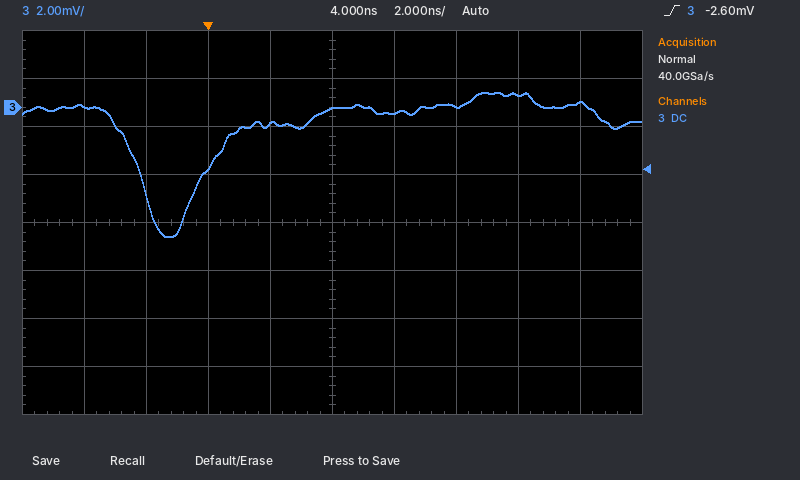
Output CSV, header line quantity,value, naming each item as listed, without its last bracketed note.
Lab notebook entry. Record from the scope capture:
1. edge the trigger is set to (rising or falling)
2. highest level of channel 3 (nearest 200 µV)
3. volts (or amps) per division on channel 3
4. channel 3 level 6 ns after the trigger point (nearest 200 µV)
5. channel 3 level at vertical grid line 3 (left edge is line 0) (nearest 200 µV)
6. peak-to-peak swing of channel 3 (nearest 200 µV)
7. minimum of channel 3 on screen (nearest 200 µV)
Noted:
quantity,value
edge the trigger is set to,rising
highest level of channel 3,600 µV
volts (or amps) per division on channel 3,2 mV
channel 3 level 6 ns after the trigger point,-200 µV
channel 3 level at vertical grid line 3 (left edge is line 0),-2.6 mV
peak-to-peak swing of channel 3,6.0 mV
minimum of channel 3 on screen,-5.4 mV
